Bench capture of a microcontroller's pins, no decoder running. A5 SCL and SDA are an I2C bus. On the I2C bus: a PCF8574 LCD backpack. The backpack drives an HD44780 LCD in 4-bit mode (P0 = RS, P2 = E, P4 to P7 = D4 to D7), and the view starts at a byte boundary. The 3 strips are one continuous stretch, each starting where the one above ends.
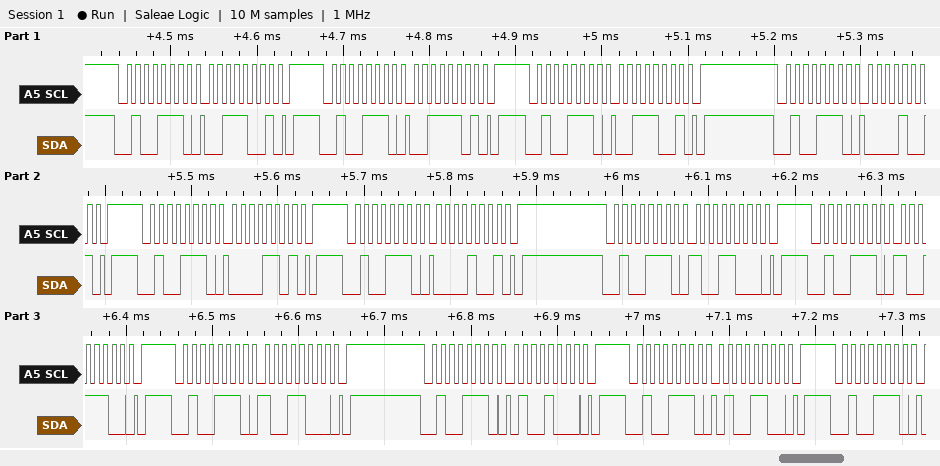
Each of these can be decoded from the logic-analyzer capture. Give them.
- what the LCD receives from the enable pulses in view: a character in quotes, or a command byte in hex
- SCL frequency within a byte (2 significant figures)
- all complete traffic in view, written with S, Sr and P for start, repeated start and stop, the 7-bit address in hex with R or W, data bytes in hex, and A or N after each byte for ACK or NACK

'0'
100 kHz
S 27W A 39 A P S 27W A 3D A P S 27W A 39 A P S 27W A 09 A P S 27W A 0D A P S 27W A 09 A P S 27W A 98 A P S 27W A 9C A P S 27W A 98 A P S 27W A 48 A P S 27W A 4C A P S 27W A
